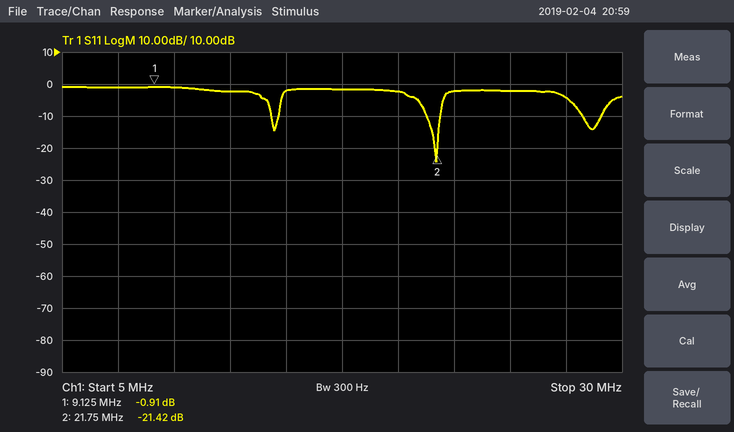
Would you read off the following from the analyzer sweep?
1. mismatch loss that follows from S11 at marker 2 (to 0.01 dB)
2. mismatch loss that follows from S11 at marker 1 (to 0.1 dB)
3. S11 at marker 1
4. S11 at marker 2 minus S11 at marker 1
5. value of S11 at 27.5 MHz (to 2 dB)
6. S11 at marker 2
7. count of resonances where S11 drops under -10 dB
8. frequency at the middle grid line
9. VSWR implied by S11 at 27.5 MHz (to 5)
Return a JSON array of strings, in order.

["0.03 dB", "7.2 dB", "-0.91 dB", "-20.51 dB", "-4 dB", "-21.42 dB", "3", "17.5 MHz", "5"]
